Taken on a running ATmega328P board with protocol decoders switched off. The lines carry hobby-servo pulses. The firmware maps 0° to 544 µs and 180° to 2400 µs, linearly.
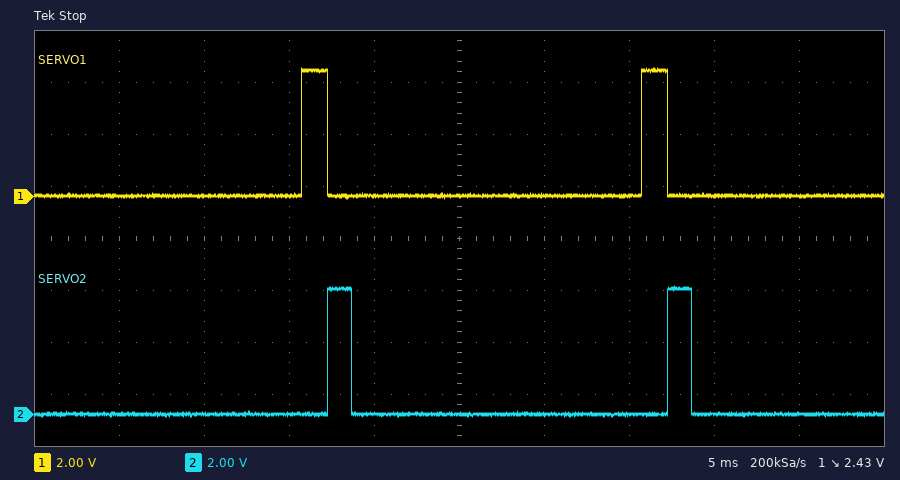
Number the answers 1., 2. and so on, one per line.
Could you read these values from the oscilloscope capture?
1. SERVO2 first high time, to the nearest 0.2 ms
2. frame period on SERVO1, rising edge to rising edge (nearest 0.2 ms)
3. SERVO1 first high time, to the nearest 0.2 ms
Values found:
1. 1.4 ms
2. 20.0 ms
3. 1.6 ms
